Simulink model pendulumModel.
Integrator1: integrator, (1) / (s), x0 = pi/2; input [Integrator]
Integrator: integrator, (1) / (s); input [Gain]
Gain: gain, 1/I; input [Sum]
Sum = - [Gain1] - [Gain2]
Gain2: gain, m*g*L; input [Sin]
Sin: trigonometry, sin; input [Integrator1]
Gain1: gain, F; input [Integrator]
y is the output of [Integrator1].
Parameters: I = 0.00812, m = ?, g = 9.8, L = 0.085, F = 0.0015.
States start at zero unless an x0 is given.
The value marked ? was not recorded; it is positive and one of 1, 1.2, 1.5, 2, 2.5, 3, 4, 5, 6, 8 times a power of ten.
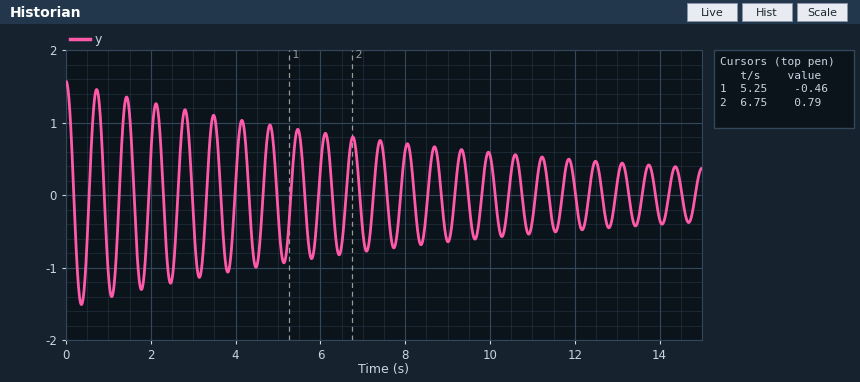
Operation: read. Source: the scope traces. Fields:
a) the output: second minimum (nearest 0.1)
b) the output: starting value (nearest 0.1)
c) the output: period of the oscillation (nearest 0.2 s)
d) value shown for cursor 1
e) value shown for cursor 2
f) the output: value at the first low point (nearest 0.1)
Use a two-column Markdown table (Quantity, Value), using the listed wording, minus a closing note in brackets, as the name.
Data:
| Quantity | Value |
|---|---|
| the output: second minimum | -1.4 |
| the output: starting value | 1.6 |
| the output: period of the oscillation | 0.8 s |
| value shown for cursor 1 | -0.46 |
| value shown for cursor 2 | 0.79 |
| the output: value at the first low point | -1.5 |
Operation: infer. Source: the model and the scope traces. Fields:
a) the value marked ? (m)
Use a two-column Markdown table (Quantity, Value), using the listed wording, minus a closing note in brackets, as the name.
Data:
| Quantity | Value |
|---|---|
| the value marked ? | 1 |
